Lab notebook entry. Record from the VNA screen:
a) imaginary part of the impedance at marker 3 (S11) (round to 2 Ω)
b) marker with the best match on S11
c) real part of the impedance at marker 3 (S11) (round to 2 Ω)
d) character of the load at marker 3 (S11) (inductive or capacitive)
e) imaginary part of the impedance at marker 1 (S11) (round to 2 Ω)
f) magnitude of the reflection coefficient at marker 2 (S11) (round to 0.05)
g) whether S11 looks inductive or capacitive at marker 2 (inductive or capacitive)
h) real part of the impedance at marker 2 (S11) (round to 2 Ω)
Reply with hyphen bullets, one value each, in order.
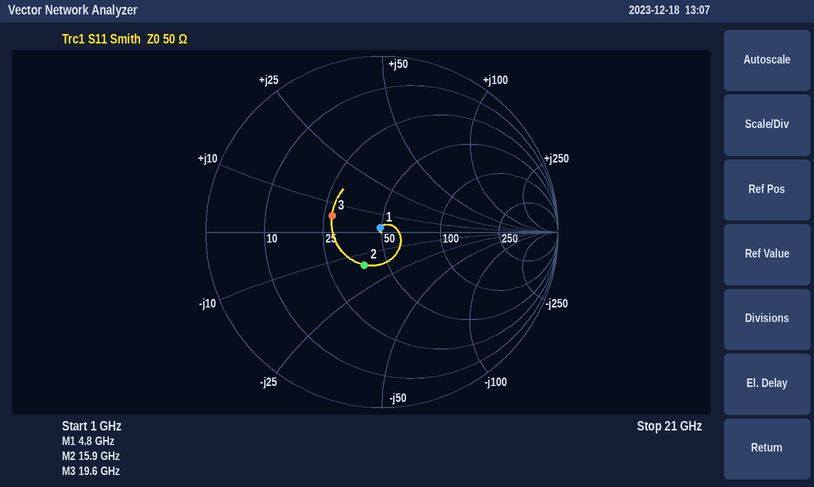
- +6 Ω
- marker 1
- 28 Ω
- inductive
- +2 Ω
- 0.20
- capacitive
- 38 Ω
